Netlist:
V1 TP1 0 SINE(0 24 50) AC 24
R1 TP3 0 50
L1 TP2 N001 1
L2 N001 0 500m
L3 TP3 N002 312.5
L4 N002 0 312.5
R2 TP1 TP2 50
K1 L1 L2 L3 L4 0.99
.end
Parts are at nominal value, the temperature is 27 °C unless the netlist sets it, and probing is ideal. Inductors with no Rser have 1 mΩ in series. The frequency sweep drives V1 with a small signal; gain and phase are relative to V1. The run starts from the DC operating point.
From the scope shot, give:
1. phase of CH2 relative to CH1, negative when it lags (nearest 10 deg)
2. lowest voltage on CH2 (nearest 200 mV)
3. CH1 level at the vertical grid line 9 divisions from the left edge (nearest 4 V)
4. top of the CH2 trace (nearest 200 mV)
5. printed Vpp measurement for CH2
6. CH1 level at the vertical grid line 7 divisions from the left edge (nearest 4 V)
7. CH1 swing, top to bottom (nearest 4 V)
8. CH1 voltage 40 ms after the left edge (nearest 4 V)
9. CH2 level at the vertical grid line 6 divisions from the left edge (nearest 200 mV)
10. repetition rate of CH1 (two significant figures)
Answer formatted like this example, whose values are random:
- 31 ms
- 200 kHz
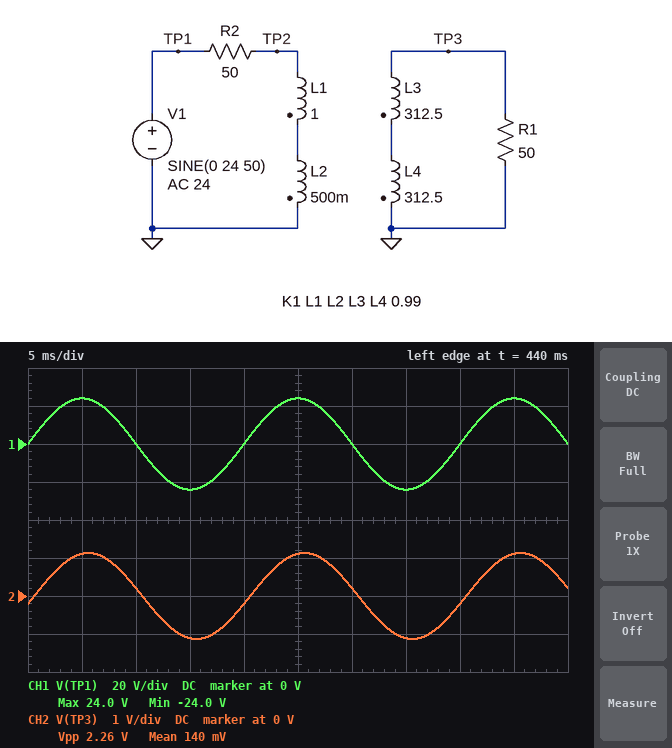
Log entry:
- -10 deg
- -1.2 V
- 24 V
- 1.2 V
- 2.26 V
- -24 V
- 48 V
- 0 V
- 200 mV
- 50 Hz
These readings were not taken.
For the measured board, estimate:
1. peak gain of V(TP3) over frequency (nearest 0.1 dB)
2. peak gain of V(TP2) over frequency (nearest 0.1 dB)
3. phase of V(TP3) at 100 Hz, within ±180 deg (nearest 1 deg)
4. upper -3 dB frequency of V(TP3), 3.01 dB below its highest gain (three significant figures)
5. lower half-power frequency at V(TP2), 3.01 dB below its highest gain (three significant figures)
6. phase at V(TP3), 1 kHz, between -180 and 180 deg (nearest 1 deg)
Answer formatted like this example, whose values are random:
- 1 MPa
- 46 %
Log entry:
- -26.4 dB
- 0 dB
- -20 deg
- 270 Hz
- 270 Hz
- -75 deg
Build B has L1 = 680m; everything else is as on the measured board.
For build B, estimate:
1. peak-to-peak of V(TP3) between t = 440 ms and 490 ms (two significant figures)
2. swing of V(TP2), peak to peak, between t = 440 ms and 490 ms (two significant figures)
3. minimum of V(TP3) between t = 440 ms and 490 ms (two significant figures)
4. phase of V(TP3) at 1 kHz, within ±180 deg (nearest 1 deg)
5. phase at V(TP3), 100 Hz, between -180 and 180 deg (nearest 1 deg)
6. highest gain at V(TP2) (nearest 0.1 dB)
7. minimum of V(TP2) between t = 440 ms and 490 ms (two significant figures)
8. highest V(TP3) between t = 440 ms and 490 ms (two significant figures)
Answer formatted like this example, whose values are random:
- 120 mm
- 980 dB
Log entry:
- 2.0 V
- 7.0 V
- -1.0 V
- -71 deg
- -16 deg
- 0 dB
- -3.5 V
- 1.0 V
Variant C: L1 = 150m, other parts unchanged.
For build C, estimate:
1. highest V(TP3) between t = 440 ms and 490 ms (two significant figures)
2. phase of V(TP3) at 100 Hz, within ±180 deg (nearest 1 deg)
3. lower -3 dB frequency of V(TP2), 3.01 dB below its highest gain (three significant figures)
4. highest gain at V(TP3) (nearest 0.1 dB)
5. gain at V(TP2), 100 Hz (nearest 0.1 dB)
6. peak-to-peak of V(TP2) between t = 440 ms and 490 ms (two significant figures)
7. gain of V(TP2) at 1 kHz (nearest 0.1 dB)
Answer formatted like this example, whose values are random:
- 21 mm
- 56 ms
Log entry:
- 740 mV
- -9 deg
- 639 Hz
- -30.2 dB
- -16.2 dB
- 3.7 V
- -1.5 dB
